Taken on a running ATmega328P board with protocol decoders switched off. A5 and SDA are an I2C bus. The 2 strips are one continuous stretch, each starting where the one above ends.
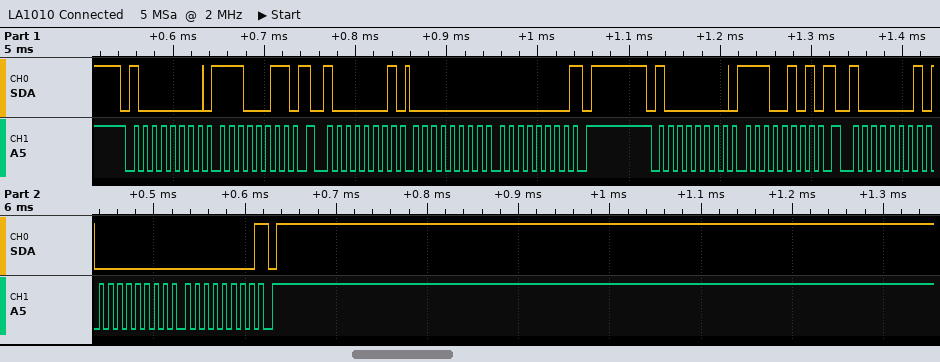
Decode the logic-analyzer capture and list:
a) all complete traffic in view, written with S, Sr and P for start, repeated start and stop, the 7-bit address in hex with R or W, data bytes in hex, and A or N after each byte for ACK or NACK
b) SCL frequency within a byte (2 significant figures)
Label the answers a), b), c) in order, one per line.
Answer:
a) S 40W A E3 A Sr 40R A 00 A 00 N P S 40W A E5 A Sr 40R A 00 A 00 N P
b) 100 kHz
